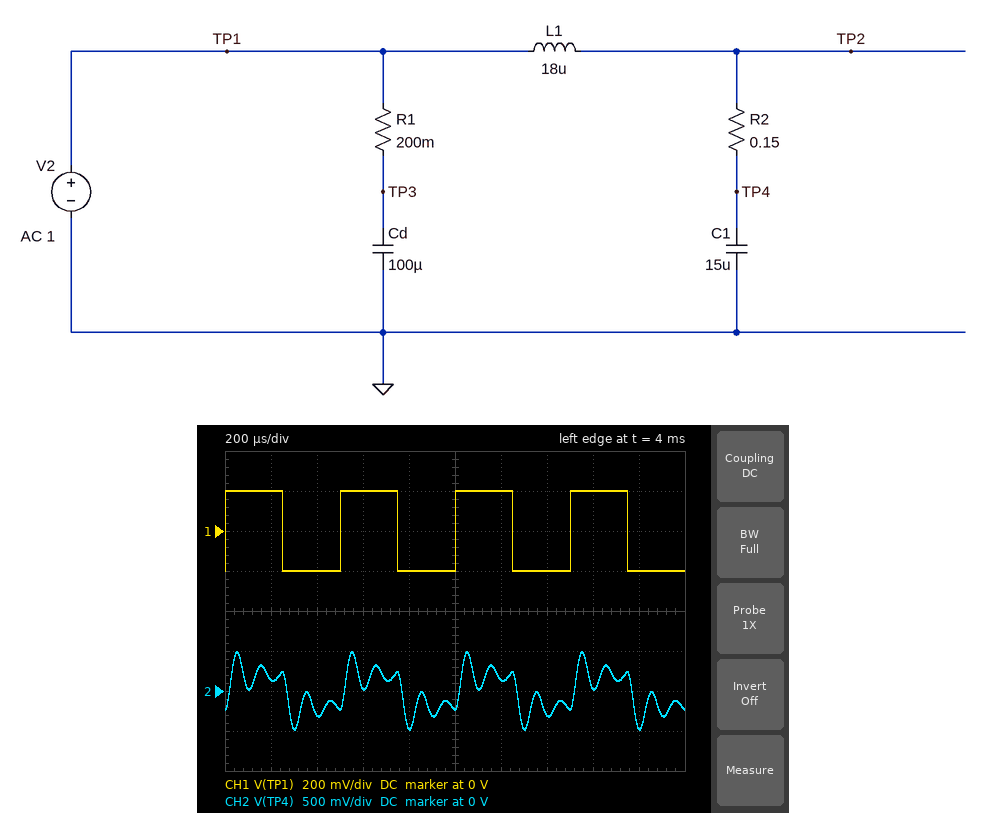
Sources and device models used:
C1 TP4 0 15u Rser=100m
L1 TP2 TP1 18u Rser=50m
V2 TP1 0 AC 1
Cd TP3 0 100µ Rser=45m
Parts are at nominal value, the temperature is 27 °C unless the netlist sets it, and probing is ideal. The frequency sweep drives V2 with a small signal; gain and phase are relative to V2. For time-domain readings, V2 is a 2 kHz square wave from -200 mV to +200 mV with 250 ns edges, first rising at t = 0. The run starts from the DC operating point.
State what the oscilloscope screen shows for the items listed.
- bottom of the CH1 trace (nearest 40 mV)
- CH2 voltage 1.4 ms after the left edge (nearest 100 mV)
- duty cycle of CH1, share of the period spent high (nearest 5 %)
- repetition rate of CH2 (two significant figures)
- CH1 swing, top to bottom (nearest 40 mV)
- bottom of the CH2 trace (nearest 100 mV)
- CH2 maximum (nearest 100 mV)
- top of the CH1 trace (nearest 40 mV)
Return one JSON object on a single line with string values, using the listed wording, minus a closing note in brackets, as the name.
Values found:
{"bottom of the CH1 trace": "-200 mV", "CH2 voltage 1.4 ms after the left edge": "-300 mV", "duty cycle of CH1, share of the period spent high": "50 %", "repetition rate of CH2": "2.0 kHz", "CH1 swing, top to bottom": "400 mV", "bottom of the CH2 trace": "-500 mV", "CH2 maximum": "500 mV", "top of the CH1 trace": "200 mV"}
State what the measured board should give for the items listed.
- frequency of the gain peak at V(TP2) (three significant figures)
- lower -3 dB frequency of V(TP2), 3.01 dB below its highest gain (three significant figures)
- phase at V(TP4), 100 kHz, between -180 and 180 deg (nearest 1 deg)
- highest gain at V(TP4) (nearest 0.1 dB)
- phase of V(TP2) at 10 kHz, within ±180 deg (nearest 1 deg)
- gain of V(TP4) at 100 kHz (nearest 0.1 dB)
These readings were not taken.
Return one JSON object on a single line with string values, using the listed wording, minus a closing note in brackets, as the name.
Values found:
{"frequency of the gain peak at V(TP2)": "9.51 kHz", "lower -3 dB frequency of V(TP2), 3.01 dB below its highest gain": "8.07 kHz", "phase at V(TP4), 100 kHz, between -180 and 180 deg": "-135 deg", "highest gain at V(TP4)": "11.4 dB", "phase of V(TP2) at 10 kHz, within ±180 deg": "-90 deg", "gain of V(TP4) at 100 kHz": "-37.7 dB"}
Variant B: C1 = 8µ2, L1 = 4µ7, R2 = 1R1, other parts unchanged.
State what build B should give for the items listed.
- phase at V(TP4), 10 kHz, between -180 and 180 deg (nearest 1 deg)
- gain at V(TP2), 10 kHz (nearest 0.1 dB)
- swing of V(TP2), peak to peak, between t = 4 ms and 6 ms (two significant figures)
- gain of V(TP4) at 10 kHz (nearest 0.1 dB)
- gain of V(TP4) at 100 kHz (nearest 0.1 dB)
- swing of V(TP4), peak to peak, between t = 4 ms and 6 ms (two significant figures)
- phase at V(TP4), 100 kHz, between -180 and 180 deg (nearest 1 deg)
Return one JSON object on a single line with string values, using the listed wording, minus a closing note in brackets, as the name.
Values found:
{"phase at V(TP4), 10 kHz, between -180 and 180 deg": "-34 deg", "gain at V(TP2), 10 kHz": "0.9 dB", "swing of V(TP2), peak to peak, between t = 4 ms and 6 ms": "530 mV", "gain of V(TP4) at 10 kHz": "-0.5 dB", "gain of V(TP4) at 100 kHz": "-22.8 dB", "swing of V(TP4), peak to peak, between t = 4 ms and 6 ms": "410 mV", "phase at V(TP4), 100 kHz, between -180 and 180 deg": "-128 deg"}
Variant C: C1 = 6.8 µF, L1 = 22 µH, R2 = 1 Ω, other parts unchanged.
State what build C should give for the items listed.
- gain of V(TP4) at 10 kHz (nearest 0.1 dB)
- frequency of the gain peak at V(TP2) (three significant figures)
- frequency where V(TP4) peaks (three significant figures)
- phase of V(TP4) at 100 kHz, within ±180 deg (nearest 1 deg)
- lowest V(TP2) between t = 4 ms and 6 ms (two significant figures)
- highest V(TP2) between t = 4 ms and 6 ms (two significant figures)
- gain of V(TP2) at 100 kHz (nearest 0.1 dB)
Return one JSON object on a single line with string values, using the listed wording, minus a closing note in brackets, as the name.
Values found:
{"gain of V(TP4) at 10 kHz": "3.9 dB", "frequency of the gain peak at V(TP2)": "12.0 kHz", "frequency where V(TP4) peaks": "11.6 kHz", "phase of V(TP4) at 100 kHz, within ±180 deg": "-152 deg", "lowest V(TP2) between t = 4 ms and 6 ms": "-370 mV", "highest V(TP2) between t = 4 ms and 6 ms": "370 mV", "gain of V(TP2) at 100 kHz": "-21.7 dB"}
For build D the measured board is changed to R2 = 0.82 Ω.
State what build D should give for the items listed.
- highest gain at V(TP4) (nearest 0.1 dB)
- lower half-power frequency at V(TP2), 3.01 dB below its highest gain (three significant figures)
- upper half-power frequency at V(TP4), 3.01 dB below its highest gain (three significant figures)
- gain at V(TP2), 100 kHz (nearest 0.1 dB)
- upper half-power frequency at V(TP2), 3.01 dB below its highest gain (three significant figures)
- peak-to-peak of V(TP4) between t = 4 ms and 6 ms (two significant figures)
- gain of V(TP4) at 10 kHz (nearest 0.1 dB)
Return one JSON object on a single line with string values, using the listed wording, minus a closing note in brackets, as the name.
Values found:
{"highest gain at V(TP4)": "2.0 dB", "lower half-power frequency at V(TP2), 3.01 dB below its highest gain": "2.84 kHz", "upper half-power frequency at V(TP4), 3.01 dB below its highest gain": "11.5 kHz", "gain at V(TP2), 100 kHz": "-21.7 dB", "upper half-power frequency at V(TP2), 3.01 dB below its highest gain": "12.7 kHz", "peak-to-peak of V(TP4) between t = 4 ms and 6 ms": "570 mV", "gain of V(TP4) at 10 kHz": "0.8 dB"}
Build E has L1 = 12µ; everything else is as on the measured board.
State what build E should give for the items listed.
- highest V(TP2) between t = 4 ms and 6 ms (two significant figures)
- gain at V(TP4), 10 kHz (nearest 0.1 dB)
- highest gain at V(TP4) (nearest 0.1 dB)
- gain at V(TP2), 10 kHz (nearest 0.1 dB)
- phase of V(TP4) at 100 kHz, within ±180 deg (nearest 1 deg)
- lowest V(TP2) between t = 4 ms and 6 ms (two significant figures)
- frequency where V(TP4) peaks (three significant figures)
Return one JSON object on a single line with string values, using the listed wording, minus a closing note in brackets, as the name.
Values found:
{"highest V(TP2) between t = 4 ms and 6 ms": "440 mV", "gain at V(TP4), 10 kHz": "7.9 dB", "highest gain at V(TP4)": "9.7 dB", "gain at V(TP2), 10 kHz": "8.1 dB", "phase of V(TP4) at 100 kHz, within ±180 deg": "-134 deg", "lowest V(TP2) between t = 4 ms and 6 ms": "-440 mV", "frequency where V(TP4) peaks": "11.5 kHz"}
